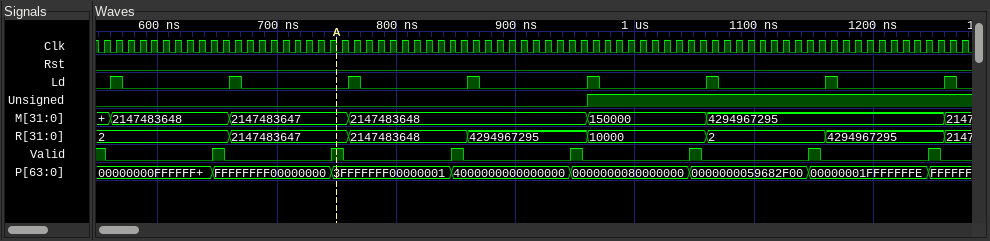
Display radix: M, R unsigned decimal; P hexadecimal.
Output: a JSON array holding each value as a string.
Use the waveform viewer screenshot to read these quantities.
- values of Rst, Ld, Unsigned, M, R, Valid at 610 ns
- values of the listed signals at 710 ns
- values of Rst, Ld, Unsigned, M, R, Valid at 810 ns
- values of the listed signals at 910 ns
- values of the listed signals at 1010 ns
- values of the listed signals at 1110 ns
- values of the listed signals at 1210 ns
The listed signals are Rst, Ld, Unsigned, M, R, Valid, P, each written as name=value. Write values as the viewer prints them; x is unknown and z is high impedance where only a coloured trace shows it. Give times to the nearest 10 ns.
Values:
["Rst=0, Ld=0, Unsigned=0, M=2147483648, R=2, Valid=0", "Rst=0, Ld=0, Unsigned=0, M=2147483647, R=2147483647, Valid=0, P=FFFFFFFF00000000", "Rst=0, Ld=0, Unsigned=0, M=2147483648, R=2147483648, Valid=0", "Rst=0, Ld=0, Unsigned=0, M=2147483648, R=4294967295, Valid=0, P=4000000000000000", "Rst=0, Ld=0, Unsigned=1, M=150000, R=10000, Valid=0, P=0000000080000000", "Rst=0, Ld=0, Unsigned=1, M=4294967295, R=2, Valid=0, P=0000000059682F00", "Rst=0, Ld=0, Unsigned=1, M=4294967295, R=4294967295, Valid=0, P=00000001FFFFFFFE"]
